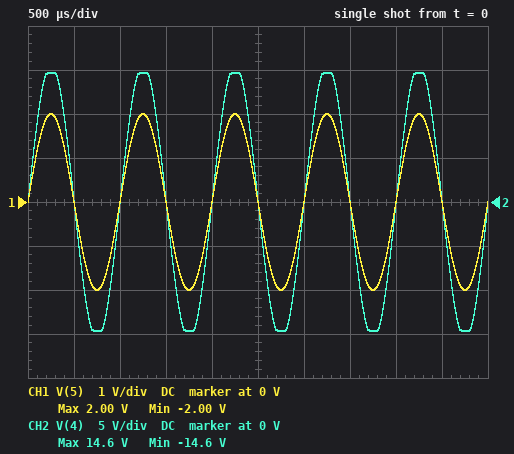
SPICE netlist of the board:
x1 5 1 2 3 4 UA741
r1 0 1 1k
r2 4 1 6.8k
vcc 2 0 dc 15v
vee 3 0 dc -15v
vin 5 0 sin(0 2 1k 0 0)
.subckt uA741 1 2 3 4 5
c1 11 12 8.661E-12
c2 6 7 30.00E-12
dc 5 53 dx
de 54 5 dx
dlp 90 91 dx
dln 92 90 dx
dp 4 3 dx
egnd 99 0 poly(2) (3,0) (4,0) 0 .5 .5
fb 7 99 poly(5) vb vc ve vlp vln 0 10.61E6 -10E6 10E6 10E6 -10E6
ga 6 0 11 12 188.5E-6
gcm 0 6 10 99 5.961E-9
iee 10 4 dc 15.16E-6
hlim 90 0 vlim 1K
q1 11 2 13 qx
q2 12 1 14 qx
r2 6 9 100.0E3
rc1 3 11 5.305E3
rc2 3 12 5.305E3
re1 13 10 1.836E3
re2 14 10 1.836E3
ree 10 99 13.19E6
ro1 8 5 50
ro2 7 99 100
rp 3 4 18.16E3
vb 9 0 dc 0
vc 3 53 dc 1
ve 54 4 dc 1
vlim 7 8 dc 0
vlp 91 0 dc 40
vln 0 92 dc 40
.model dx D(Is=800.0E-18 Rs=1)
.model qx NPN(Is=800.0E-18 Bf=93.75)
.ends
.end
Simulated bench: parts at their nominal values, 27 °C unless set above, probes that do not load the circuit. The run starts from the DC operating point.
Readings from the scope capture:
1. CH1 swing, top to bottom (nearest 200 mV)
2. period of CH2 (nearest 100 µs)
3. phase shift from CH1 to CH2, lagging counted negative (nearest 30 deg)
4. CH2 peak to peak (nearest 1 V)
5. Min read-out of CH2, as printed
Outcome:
4.0 V
1.0 ms
0 deg
29 V
-14.6 V
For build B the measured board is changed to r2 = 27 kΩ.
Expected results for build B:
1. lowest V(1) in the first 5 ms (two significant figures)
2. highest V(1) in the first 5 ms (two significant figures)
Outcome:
-520 mV
520 mV
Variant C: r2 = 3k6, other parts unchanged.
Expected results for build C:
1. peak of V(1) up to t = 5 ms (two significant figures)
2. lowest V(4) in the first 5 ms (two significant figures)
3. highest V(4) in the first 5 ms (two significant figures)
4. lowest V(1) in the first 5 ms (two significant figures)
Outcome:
2.0 V
-9.2 V
9.2 V
-2.0 V
